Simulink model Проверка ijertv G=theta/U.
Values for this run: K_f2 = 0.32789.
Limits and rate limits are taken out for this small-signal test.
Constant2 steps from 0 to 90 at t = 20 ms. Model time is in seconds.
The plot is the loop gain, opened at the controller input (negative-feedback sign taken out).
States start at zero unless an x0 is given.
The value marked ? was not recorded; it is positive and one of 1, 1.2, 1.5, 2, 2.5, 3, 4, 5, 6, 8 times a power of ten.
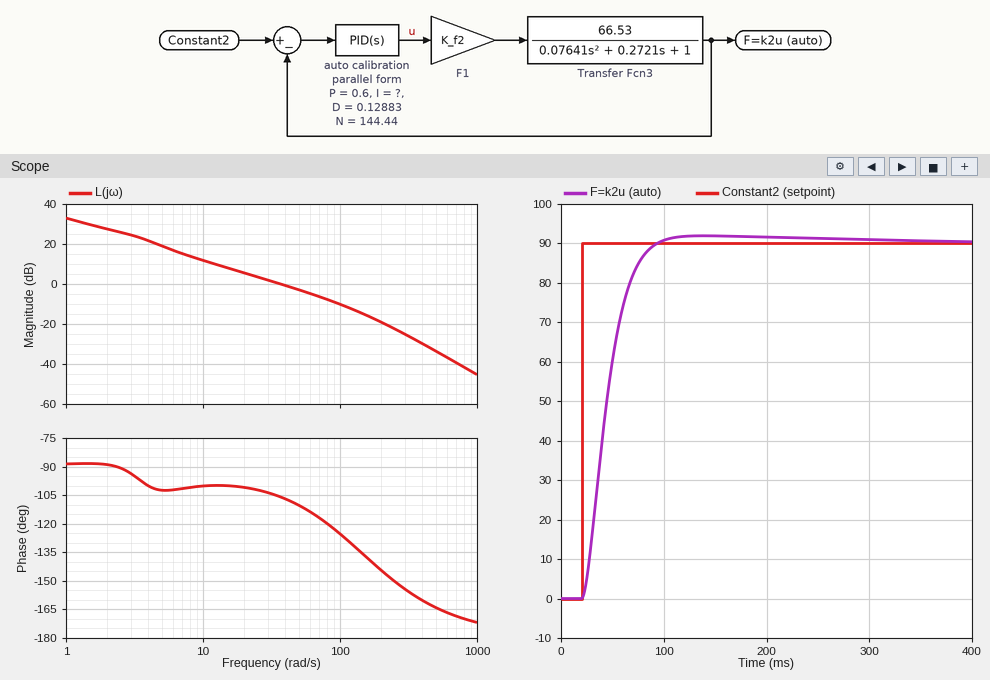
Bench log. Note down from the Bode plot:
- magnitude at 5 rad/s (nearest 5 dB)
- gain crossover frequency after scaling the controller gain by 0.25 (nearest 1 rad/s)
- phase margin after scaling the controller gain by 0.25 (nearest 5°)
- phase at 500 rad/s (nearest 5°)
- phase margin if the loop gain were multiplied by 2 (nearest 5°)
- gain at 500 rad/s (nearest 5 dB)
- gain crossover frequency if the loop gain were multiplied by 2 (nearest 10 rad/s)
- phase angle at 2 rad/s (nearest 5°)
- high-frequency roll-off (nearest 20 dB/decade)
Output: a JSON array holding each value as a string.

["20 dB", "10 rad/s", "80°", "-165°", "65°", "-35 dB", "70 rad/s", "-90°", "-40 dB/decade"]
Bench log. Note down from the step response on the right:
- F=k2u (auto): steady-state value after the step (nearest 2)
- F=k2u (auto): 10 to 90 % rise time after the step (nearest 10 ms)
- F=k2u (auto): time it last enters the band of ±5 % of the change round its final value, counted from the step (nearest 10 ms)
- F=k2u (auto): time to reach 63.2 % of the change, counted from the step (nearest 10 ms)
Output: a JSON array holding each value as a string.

["90", "40 ms", "60 ms", "30 ms"]
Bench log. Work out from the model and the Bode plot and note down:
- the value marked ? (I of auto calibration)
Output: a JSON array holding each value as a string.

["2"]
